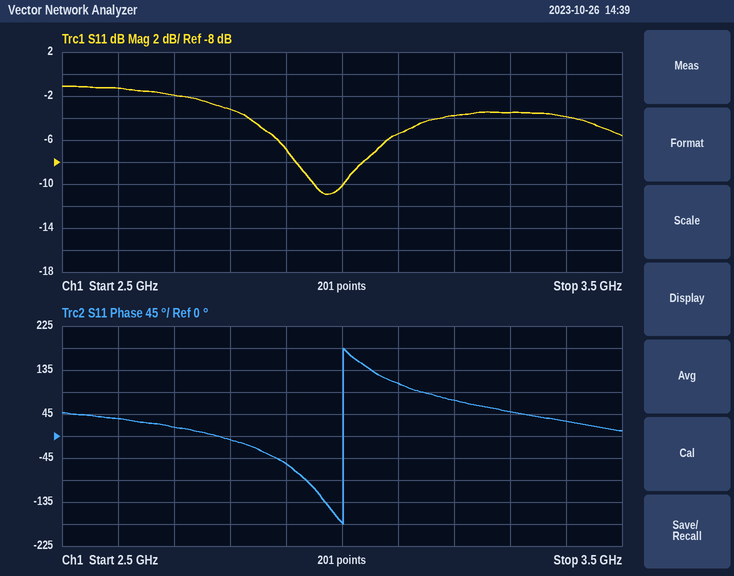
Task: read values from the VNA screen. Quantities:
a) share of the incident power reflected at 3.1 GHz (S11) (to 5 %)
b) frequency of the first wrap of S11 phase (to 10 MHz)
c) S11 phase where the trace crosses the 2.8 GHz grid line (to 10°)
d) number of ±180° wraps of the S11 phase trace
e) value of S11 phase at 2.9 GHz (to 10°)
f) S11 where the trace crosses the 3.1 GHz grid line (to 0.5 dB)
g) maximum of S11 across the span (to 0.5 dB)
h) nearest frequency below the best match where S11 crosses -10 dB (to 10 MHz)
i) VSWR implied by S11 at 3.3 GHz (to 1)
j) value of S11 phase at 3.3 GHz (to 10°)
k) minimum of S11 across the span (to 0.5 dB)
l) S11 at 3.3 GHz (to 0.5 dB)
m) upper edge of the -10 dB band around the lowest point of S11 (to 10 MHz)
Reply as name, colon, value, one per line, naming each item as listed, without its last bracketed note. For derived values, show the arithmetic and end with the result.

share of the incident power reflected at 3.1 GHz (S11): 10^(-5.5/10) ≈ 28.2 %, so 30 % to the nearest 5 %
frequency of the first wrap of S11 phase: 3.00 GHz
S11 phase where the trace crosses the 2.8 GHz grid line: -10°
number of ±180° wraps of the S11 phase trace: 1
value of S11 phase at 2.9 GHz: -60°
S11 where the trace crosses the 3.1 GHz grid line: -5.5 dB
maximum of S11 across the span: -1.0 dB
nearest frequency below the best match where S11 crosses -10 dB: 2.95 GHz
VSWR implied by S11 at 3.3 GHz: |Γ| = 10^(-3.5/20) = 0.6683; VSWR = (1 + 0.6683)/(1 − 0.6683) ≈ 5
value of S11 phase at 3.3 GHz: 50°
minimum of S11 across the span: -11.0 dB
S11 at 3.3 GHz: -3.5 dB
upper edge of the -10 dB band around the lowest point of S11: 3.00 GHz
